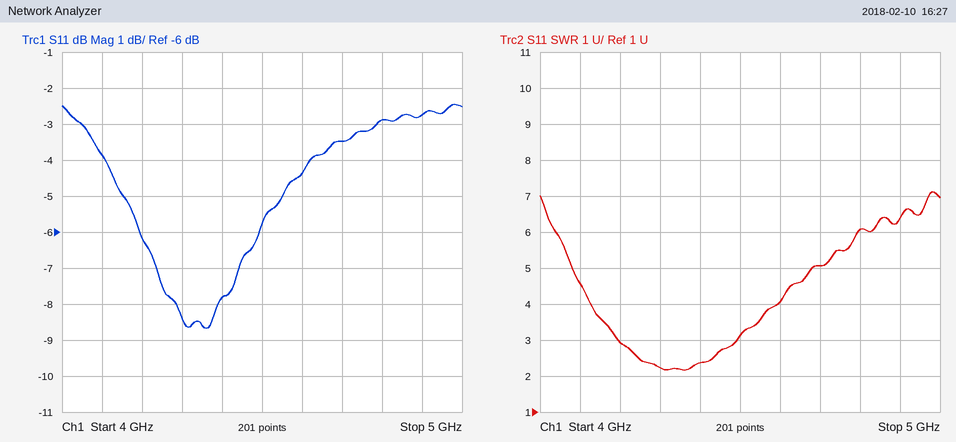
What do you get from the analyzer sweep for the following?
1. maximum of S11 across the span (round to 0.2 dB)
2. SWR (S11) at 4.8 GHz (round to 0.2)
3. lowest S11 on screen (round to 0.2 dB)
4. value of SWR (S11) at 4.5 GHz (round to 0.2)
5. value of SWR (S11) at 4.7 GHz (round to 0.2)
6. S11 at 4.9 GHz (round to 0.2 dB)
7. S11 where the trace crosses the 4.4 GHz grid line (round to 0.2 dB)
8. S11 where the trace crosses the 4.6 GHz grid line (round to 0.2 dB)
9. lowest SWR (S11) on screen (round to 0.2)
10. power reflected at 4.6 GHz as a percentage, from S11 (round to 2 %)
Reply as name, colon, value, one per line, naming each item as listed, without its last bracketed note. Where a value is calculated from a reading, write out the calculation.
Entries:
maximum of S11 across the span: -2.4 dB
SWR (S11) at 4.8 GHz: 6.0
lowest S11 on screen: -8.6 dB
value of SWR (S11) at 4.5 GHz: 3.2
value of SWR (S11) at 4.7 GHz: 5.0
S11 at 4.9 GHz: -2.8 dB
S11 where the trace crosses the 4.4 GHz grid line: -7.8 dB
S11 where the trace crosses the 4.6 GHz grid line: -4.4 dB
lowest SWR (S11) on screen: 2.2
power reflected at 4.6 GHz as a percentage, from S11: 10^(-4.4/10) ≈ 36 %
